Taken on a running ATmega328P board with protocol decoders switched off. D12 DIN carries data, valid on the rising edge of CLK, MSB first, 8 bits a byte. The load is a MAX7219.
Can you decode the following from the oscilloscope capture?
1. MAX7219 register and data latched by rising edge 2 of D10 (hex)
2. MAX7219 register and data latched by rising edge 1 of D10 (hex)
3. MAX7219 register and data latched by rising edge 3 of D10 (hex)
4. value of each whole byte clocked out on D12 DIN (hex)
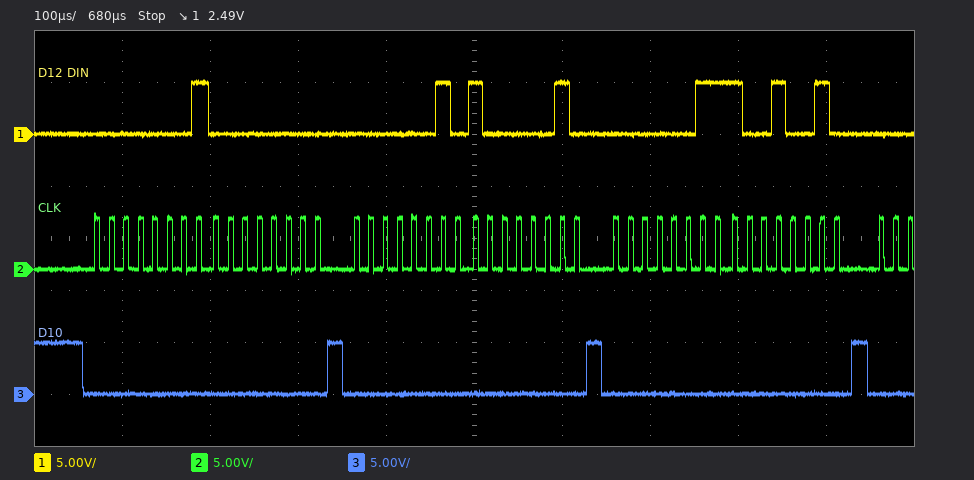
register 0x2, data 0x82
register 0x1, data 0x00
register 0x3, data 0x92
0x01 0x00 0x02 0x82 0x03 0x92
